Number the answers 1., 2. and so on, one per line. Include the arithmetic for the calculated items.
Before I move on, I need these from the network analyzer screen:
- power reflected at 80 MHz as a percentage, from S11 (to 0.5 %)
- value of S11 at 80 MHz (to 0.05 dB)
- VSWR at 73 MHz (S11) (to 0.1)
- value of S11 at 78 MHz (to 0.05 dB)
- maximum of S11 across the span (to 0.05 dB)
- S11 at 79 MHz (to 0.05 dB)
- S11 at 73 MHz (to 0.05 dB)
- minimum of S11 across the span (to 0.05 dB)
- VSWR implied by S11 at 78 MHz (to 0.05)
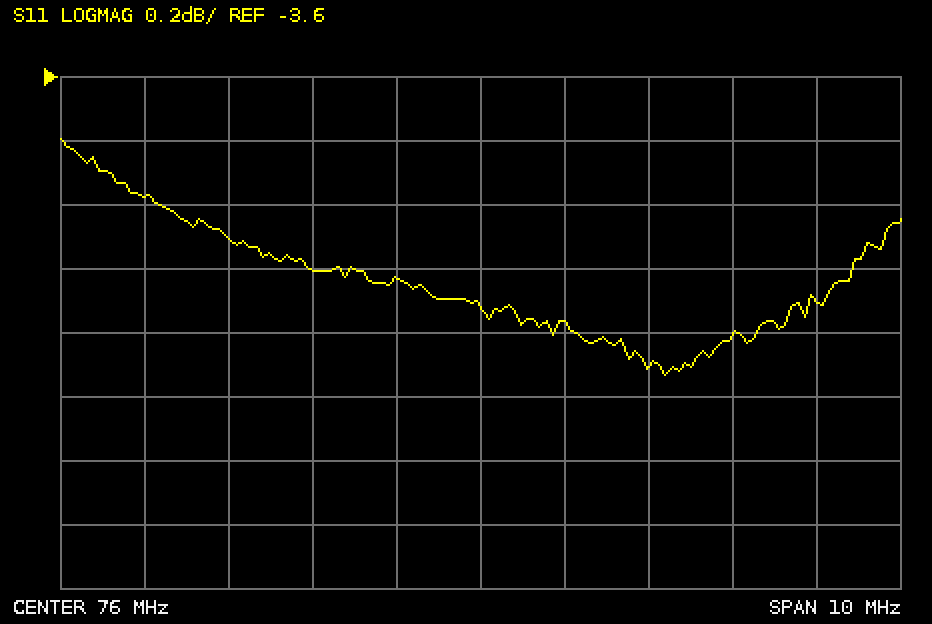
1. 10^(-4.3/10) ≈ 37.2 %, so 37.0 % to the nearest 0.5 %
2. -4.30 dB
3. |Γ| = 10^(-4.1/20) = 0.6237; VSWR = (1 + 0.6237)/(1 − 0.6237) ≈ 4.3
4. -4.50 dB
5. -3.80 dB
6. -4.40 dB
7. -4.10 dB
8. -4.55 dB
9. |Γ| = 10^(-4.5/20) = 0.5957; VSWR = (1 + 0.5957)/(1 − 0.5957) ≈ 3.95
